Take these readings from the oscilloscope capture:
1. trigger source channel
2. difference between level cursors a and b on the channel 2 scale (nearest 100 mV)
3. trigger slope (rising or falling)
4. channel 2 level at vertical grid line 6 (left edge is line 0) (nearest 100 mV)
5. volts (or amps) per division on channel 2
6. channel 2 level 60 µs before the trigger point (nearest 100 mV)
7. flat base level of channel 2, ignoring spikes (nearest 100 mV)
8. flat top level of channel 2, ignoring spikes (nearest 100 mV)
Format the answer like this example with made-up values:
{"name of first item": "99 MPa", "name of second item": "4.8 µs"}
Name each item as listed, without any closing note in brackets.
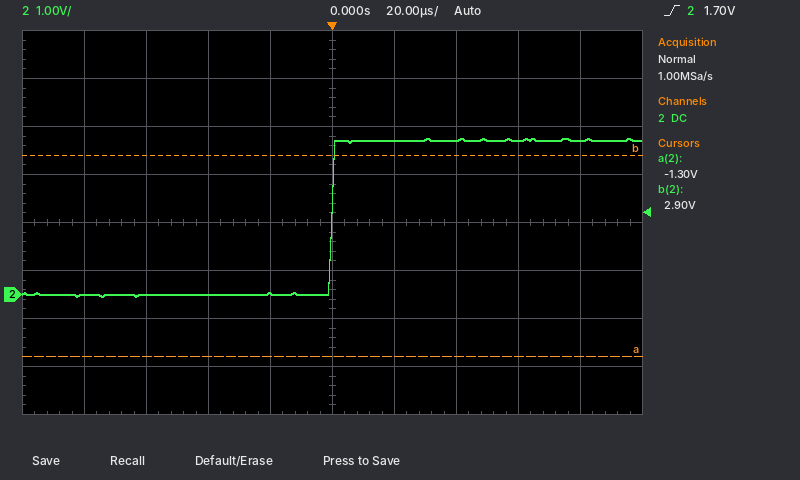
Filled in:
{"trigger source channel": "channel 2", "difference between level cursors a and b on the channel 2 scale": "4.2 V", "trigger slope": "rising", "channel 2 level at vertical grid line 6 (left edge is line 0)": "3.2 V", "volts (or amps) per division on channel 2": "1 V", "channel 2 level 60 µs before the trigger point": "0.0 V", "flat base level of channel 2, ignoring spikes": "0.0 V", "flat top level of channel 2, ignoring spikes": "3.2 V"}
